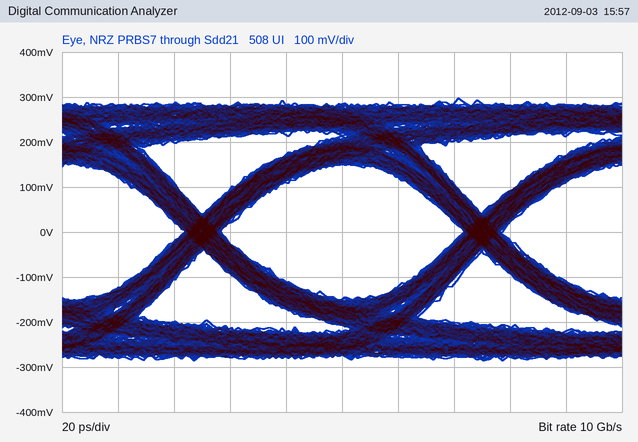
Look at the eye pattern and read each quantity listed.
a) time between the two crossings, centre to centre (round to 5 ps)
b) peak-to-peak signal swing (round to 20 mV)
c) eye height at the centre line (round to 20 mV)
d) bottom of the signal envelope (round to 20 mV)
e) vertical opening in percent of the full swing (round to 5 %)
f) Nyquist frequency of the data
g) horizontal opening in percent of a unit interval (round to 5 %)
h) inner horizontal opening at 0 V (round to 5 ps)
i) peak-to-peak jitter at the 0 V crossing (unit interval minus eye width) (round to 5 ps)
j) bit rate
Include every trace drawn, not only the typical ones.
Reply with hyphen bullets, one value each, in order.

- 100 ps
- 580 mV
- 300 mV
- -280 mV
- 50 %
- 5 GHz
- 85 %
- 85 ps
- 15 ps
- 10 Gb/s
